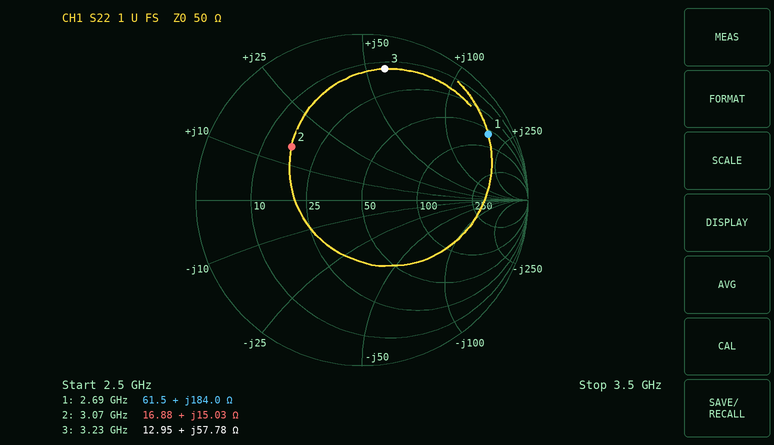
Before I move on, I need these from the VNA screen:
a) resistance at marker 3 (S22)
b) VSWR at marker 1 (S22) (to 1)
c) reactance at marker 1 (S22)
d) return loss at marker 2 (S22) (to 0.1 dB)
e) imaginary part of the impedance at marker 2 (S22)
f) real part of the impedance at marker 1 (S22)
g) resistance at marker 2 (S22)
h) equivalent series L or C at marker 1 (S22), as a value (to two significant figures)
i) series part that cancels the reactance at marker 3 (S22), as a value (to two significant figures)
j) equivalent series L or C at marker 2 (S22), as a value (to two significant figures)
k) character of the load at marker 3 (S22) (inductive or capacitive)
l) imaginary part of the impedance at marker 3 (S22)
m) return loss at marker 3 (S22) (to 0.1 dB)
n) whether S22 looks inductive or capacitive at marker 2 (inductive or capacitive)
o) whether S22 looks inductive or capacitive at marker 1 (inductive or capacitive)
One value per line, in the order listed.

12.95 Ω
13
+184.0 Ω
5.5 dB
+15.03 Ω
61.5 Ω
16.88 Ω
11 nH
850 fF
780 pH
inductive
+57.78 Ω
1.9 dB
inductive
inductive
